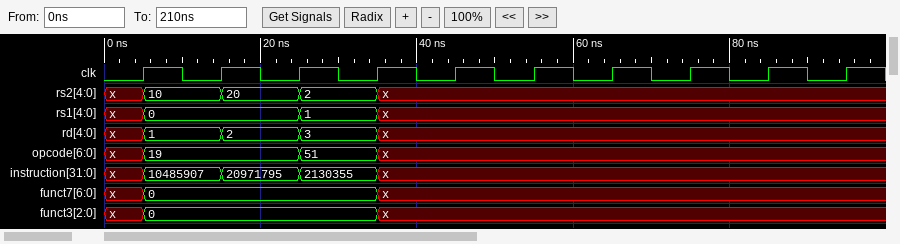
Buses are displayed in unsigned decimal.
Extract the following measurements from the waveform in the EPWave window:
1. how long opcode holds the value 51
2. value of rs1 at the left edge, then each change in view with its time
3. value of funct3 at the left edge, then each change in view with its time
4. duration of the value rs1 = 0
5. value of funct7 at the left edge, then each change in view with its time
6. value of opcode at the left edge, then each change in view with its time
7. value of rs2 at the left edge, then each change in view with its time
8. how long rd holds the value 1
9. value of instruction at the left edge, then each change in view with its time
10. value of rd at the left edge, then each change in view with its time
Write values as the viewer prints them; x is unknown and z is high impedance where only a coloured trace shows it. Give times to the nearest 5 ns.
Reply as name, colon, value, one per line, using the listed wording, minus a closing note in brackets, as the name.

how long opcode holds the value 51: 10 ns
value of rs1 at the left edge, then each change in view with its time: x, 0 at 5 ns, 1 at 25 ns, x at 35 ns
value of funct3 at the left edge, then each change in view with its time: x, 0 at 5 ns, x at 35 ns
duration of the value rs1 = 0: 20 ns
value of funct7 at the left edge, then each change in view with its time: x, 0 at 5 ns, x at 35 ns
value of opcode at the left edge, then each change in view with its time: x, 19 at 5 ns, 51 at 25 ns, x at 35 ns
value of rs2 at the left edge, then each change in view with its time: x, 10 at 5 ns, 20 at 15 ns, 2 at 25 ns, x at 35 ns
how long rd holds the value 1: 10 ns
value of instruction at the left edge, then each change in view with its time: x, 10485907 at 5 ns, 20971795 at 15 ns, 2130355 at 25 ns, x at 35 ns
value of rd at the left edge, then each change in view with its time: x, 1 at 5 ns, 2 at 15 ns, 3 at 25 ns, x at 35 ns
